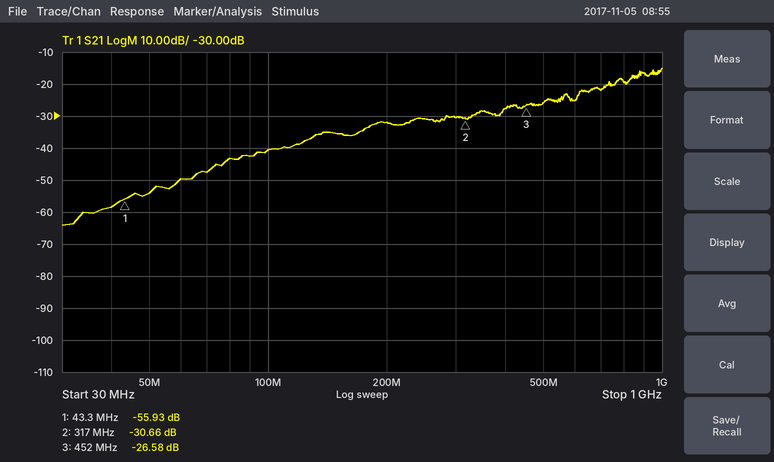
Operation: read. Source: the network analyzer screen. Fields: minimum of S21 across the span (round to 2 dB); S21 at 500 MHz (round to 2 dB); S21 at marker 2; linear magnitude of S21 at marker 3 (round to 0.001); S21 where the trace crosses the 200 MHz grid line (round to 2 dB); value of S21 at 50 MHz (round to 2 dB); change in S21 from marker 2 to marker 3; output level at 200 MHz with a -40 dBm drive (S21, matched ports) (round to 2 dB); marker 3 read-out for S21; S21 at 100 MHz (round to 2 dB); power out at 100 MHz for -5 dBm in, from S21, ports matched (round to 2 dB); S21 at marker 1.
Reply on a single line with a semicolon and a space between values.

-64 dB; -26 dB; -30.66 dB; 0.047; -32 dB; -54 dB; 4.08 dB; -72 dBm; -26.58 dB; -40 dB; -46 dBm; -55.93 dB
